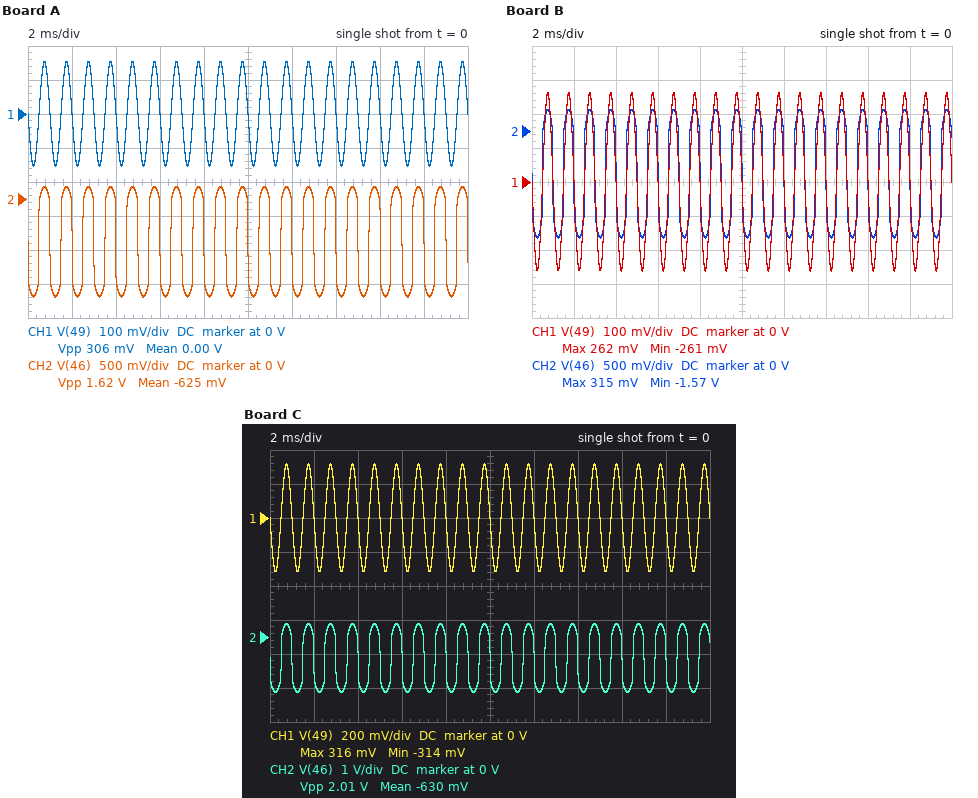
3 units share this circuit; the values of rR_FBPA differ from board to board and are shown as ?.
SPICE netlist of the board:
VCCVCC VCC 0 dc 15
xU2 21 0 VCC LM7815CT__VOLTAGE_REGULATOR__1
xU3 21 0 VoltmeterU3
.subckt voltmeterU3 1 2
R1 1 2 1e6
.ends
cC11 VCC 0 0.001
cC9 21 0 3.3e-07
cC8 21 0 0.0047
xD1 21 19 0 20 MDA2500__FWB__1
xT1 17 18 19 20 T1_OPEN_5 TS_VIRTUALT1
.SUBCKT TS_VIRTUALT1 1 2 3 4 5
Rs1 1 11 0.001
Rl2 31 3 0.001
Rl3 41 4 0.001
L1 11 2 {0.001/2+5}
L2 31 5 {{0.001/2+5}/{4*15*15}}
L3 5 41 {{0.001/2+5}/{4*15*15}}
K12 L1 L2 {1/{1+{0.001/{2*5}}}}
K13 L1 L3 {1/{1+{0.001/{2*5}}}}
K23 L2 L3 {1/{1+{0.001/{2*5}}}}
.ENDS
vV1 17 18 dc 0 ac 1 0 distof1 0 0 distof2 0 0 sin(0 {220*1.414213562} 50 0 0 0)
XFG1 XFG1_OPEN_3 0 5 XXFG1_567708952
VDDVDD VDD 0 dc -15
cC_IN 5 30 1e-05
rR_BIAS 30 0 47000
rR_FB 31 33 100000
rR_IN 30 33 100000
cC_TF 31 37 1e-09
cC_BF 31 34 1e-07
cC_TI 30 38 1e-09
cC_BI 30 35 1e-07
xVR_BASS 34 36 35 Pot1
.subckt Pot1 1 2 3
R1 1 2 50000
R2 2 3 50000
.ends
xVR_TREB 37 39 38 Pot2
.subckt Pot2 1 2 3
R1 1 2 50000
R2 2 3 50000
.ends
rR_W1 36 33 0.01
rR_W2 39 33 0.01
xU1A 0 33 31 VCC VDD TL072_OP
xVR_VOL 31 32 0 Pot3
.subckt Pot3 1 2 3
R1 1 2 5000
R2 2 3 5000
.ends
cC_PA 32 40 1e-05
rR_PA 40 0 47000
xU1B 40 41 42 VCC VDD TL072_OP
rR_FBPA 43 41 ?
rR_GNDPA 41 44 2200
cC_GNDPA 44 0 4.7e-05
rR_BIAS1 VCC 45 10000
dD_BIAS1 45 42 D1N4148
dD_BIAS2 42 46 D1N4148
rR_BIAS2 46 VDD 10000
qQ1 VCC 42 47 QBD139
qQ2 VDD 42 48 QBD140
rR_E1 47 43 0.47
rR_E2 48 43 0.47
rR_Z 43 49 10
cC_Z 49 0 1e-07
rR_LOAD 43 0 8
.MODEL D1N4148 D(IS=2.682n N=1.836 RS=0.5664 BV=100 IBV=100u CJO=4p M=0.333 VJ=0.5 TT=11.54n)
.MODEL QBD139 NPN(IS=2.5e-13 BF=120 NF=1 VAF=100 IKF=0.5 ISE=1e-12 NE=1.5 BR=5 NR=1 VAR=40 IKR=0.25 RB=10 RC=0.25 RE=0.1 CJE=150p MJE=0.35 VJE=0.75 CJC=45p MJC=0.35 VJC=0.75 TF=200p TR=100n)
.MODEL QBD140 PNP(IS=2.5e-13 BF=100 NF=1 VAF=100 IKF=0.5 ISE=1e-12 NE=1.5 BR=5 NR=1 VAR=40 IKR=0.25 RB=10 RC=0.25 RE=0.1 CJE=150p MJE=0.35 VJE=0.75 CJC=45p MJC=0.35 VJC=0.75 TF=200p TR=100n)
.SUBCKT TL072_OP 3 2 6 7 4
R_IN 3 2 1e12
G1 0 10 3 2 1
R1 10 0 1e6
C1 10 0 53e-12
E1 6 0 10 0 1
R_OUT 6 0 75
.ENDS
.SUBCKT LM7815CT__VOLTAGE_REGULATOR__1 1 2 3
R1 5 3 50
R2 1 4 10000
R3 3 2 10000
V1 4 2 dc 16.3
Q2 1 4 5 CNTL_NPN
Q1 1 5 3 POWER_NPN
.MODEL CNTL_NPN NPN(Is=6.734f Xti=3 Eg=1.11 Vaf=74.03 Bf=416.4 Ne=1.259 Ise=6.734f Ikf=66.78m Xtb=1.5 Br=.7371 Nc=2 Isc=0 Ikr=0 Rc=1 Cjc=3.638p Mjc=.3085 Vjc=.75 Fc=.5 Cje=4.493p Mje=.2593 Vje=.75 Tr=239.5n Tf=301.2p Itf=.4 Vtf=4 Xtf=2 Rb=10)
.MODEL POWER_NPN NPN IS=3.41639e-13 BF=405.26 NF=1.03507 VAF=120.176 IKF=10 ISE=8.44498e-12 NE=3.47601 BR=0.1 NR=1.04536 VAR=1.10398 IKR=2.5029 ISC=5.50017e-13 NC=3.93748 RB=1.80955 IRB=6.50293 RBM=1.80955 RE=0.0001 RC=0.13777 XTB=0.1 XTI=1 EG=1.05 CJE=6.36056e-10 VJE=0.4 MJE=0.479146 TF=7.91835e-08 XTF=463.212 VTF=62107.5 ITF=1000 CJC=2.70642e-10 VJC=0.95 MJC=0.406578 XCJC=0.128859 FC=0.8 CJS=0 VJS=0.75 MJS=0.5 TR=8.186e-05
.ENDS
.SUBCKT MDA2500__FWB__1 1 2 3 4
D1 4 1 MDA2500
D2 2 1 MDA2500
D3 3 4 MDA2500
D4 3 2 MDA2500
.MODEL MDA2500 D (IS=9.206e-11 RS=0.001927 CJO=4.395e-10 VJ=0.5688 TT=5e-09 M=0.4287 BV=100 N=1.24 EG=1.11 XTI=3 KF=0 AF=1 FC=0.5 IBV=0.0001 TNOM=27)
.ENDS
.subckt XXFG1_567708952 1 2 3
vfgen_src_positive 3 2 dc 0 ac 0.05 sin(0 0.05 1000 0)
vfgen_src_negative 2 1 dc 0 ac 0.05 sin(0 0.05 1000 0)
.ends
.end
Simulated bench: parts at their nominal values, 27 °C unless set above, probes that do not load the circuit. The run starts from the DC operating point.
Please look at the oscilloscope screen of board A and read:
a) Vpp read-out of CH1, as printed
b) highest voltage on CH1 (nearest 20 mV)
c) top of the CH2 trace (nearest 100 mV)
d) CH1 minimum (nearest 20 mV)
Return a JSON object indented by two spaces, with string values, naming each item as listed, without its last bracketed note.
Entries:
{
  "Vpp read-out of CH1, as printed": "306 mV",
  "highest voltage on CH1": "160 mV",
  "top of the CH2 trace": "200 mV",
  "CH1 minimum": "-160 mV"
}
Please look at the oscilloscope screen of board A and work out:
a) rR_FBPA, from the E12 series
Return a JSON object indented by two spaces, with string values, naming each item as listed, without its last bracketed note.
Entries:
{
  "rR_FBPA, from the E12 series": "12 kΩ"
}
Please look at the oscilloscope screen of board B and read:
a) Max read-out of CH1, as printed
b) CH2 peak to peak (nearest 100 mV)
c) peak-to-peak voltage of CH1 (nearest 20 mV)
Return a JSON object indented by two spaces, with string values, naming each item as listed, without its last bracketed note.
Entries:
{
  "Max read-out of CH1, as printed": "262 mV",
  "CH2 peak to peak": "1.9 V",
  "peak-to-peak voltage of CH1": "520 mV"
}
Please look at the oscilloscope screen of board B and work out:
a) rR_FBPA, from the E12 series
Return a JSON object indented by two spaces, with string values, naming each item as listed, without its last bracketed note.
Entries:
{
  "rR_FBPA, from the E12 series": "22 kΩ"
}
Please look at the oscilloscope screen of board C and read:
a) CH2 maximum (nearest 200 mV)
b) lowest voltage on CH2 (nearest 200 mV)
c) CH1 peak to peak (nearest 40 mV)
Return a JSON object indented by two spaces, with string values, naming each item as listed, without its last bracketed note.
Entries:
{
  "CH2 maximum": "400 mV",
  "lowest voltage on CH2": "-1.6 V",
  "CH1 peak to peak": "640 mV"
}
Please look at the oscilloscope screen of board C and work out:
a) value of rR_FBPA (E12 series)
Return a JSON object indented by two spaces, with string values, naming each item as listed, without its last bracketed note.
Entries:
{
  "value of rR_FBPA": "27 kΩ"
}
